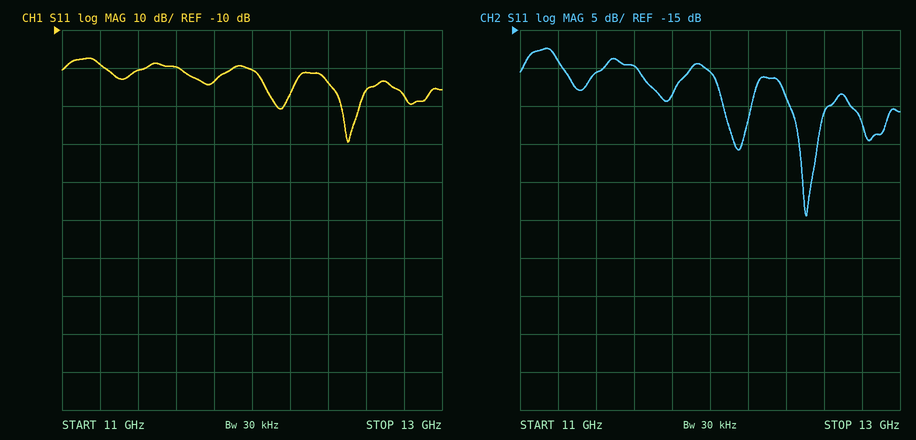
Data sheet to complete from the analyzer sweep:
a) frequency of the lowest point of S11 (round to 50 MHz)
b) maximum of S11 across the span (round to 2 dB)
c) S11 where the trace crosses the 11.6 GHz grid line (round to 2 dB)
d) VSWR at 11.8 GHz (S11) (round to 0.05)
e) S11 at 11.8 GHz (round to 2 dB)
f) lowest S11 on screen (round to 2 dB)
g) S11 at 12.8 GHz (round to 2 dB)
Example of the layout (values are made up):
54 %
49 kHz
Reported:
12.50 GHz
-18 dB
-20 dB
1.15
-24 dB
-40 dB
-28 dB
